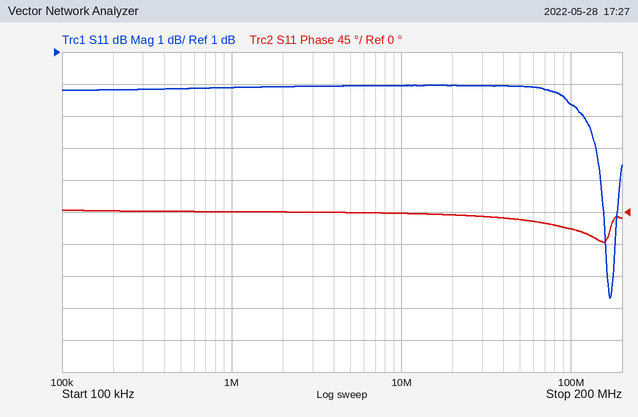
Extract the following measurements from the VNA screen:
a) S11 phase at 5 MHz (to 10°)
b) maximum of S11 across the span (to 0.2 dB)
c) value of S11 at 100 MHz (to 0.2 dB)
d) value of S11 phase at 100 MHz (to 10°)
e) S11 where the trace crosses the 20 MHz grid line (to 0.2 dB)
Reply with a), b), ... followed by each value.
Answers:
a) 0°
b) 0.0 dB
c) -0.6 dB
d) -20°
e) 0.0 dB
